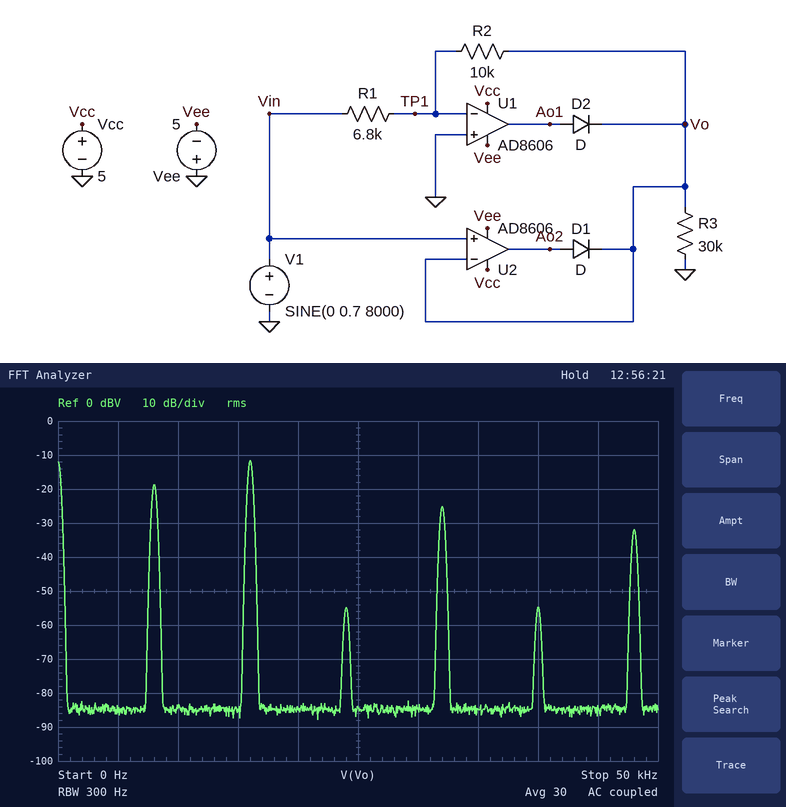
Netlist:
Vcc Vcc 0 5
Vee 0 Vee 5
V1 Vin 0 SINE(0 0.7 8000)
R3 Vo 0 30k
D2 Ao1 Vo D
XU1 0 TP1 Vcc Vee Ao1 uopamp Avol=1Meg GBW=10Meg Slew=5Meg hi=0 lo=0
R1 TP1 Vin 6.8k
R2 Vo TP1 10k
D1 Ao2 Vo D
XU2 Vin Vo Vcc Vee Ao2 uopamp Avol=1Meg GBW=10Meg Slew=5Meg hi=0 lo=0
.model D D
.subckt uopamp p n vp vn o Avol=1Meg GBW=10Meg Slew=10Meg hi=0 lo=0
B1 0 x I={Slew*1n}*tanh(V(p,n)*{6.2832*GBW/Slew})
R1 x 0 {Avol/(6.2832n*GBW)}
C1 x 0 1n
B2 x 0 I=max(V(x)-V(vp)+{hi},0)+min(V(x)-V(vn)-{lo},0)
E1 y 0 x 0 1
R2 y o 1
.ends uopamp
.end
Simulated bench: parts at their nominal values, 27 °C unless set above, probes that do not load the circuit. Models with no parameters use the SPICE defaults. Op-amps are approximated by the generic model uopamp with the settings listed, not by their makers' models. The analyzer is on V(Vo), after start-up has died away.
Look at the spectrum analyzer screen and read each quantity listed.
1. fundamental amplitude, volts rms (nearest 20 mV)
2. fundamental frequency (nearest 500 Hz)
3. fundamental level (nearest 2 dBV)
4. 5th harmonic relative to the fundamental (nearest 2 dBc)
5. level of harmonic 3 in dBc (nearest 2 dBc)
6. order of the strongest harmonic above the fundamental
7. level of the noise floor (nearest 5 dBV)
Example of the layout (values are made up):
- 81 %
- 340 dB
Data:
- 120 mV
- 8.0 kHz
- -18 dBV
- -36 dBc
- -36 dBc
- 2
- -85 dBV
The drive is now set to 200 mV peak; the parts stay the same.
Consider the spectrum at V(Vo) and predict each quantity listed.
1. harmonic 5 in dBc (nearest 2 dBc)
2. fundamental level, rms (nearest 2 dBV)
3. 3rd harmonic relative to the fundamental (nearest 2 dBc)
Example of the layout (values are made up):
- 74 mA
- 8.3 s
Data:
- -26 dBc
- -30 dBV
- -26 dBc
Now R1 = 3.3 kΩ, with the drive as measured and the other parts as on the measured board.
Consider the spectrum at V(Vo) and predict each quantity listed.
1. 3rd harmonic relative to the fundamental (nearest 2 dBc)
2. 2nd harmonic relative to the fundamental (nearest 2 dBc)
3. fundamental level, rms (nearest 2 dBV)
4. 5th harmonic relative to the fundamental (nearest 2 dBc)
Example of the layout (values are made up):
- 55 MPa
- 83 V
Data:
- -42 dBc
- -2 dBc
- -6 dBV
- -42 dBc
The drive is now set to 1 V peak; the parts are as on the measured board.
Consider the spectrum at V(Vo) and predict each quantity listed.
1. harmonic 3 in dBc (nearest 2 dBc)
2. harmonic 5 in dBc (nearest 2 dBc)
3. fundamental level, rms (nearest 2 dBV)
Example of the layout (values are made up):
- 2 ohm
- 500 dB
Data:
- -38 dBc
- -38 dBc
- -16 dBV
